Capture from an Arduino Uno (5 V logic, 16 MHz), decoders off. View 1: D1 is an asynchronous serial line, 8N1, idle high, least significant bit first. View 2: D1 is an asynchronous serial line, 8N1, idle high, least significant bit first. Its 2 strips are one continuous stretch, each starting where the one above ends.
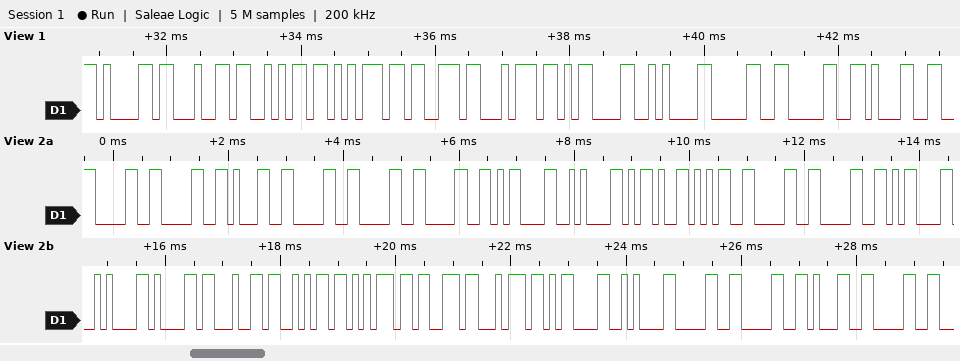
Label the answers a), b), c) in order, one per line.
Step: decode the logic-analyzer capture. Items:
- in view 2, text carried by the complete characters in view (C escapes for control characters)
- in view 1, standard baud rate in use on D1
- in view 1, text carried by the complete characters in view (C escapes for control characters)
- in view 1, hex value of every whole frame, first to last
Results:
a) "001000\r\n-500\r\nadjust\r\n0010"
b) 9600 baud
c) "adjust\r\n001"
d) 61 64 6A 75 73 74 0D 0A 30 30 31
